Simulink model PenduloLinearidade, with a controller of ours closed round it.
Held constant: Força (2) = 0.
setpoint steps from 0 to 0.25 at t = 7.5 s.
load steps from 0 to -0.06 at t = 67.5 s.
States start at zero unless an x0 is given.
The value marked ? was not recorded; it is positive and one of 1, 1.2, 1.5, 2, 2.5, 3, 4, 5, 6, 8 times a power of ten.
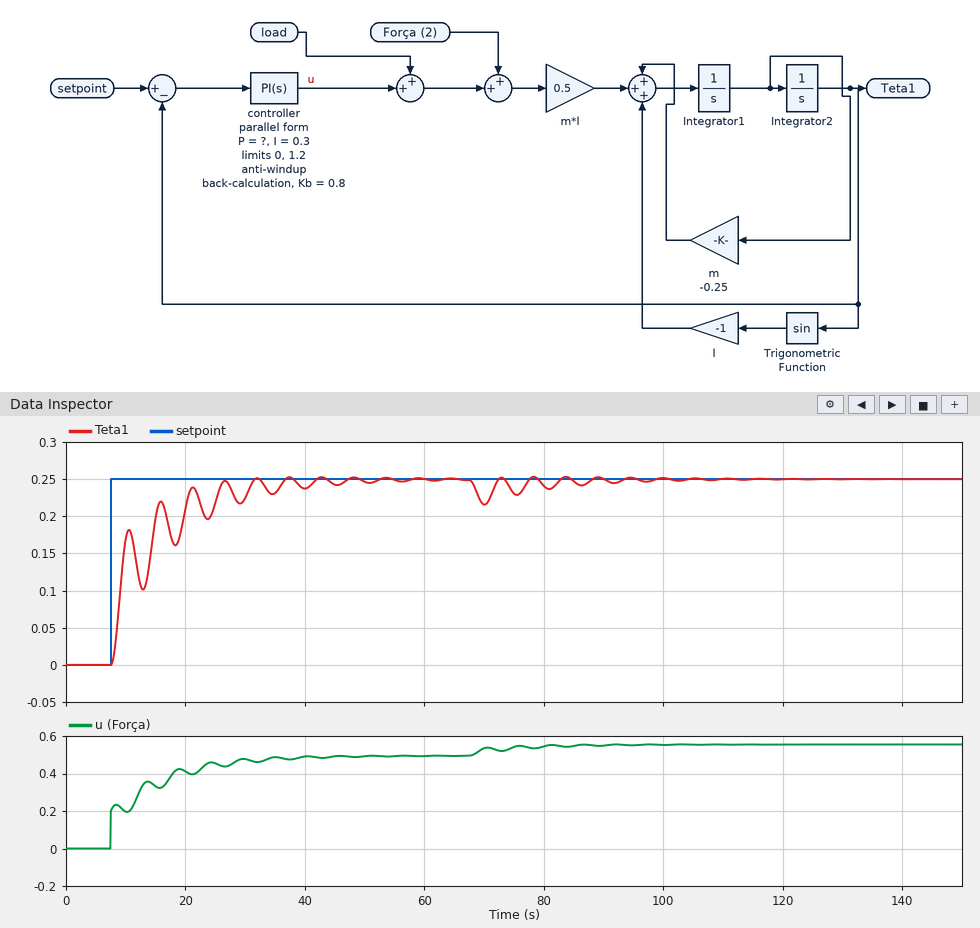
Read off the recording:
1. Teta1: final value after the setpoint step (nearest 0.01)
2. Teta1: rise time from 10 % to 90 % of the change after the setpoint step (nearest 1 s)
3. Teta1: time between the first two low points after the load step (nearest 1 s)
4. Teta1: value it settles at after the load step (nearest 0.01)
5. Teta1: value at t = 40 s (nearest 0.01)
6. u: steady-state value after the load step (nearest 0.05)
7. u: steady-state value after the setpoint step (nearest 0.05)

0.25
12 s
5 s
0.25
0.24
0.55
0.50
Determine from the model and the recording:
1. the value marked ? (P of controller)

0.8
